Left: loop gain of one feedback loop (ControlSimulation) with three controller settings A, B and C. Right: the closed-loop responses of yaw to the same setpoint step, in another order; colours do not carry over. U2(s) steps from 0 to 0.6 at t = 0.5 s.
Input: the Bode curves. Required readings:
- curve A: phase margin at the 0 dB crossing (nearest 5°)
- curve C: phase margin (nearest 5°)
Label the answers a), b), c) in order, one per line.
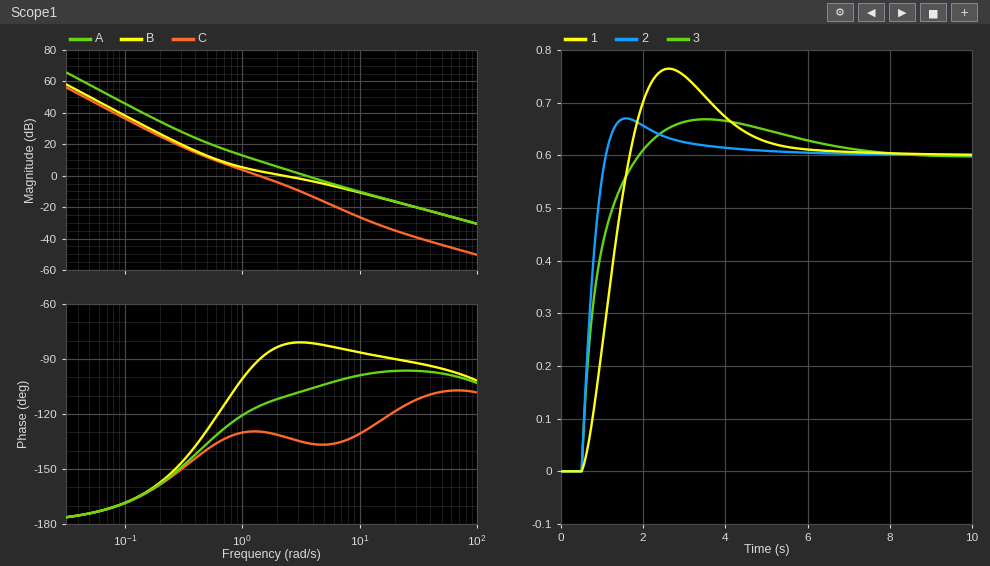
a) 75°
b) 50°
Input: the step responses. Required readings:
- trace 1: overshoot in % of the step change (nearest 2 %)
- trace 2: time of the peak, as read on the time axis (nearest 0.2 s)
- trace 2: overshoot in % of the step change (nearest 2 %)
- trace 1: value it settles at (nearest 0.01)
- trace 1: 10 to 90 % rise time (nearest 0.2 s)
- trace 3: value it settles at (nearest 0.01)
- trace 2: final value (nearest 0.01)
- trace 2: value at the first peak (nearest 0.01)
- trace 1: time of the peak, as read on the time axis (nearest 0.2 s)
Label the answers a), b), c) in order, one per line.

a) 28 %
b) 1.6 s
c) 12 %
d) 0.60
e) 0.8 s
f) 0.60
g) 0.60
h) 0.67
i) 2.6 s
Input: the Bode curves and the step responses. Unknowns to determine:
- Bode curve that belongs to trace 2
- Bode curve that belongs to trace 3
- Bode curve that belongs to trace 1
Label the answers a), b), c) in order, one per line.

a) A
b) B
c) C
